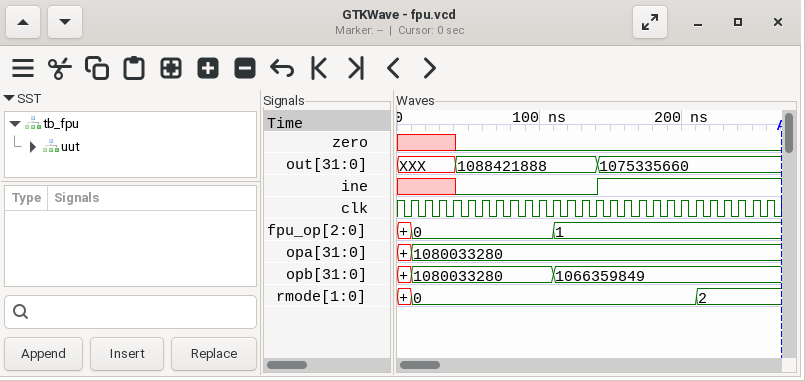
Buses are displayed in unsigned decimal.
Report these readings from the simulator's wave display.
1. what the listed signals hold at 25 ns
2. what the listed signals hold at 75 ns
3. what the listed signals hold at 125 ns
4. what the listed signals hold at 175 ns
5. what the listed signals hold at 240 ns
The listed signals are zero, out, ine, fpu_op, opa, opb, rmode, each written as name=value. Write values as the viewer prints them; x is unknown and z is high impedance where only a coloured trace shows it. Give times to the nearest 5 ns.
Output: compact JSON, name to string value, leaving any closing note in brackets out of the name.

{"what the listed signals hold at 25 ns": "zero=x, out=XXX, ine=x, fpu_op=0, opa=1080033280, opb=1080033280, rmode=0", "what the listed signals hold at 75 ns": "zero=0, out=1088421888, ine=0, fpu_op=0, opa=1080033280, opb=1080033280, rmode=0", "what the listed signals hold at 125 ns": "zero=0, out=1088421888, ine=0, fpu_op=1, opa=1080033280, opb=1066359849, rmode=0", "what the listed signals hold at 175 ns": "zero=0, out=1075335660, ine=1, fpu_op=1, opa=1080033280, opb=1066359849, rmode=0", "what the listed signals hold at 240 ns": "zero=0, out=1075335660, ine=1, fpu_op=1, opa=1080033280, opb=1066359849, rmode=2"}
